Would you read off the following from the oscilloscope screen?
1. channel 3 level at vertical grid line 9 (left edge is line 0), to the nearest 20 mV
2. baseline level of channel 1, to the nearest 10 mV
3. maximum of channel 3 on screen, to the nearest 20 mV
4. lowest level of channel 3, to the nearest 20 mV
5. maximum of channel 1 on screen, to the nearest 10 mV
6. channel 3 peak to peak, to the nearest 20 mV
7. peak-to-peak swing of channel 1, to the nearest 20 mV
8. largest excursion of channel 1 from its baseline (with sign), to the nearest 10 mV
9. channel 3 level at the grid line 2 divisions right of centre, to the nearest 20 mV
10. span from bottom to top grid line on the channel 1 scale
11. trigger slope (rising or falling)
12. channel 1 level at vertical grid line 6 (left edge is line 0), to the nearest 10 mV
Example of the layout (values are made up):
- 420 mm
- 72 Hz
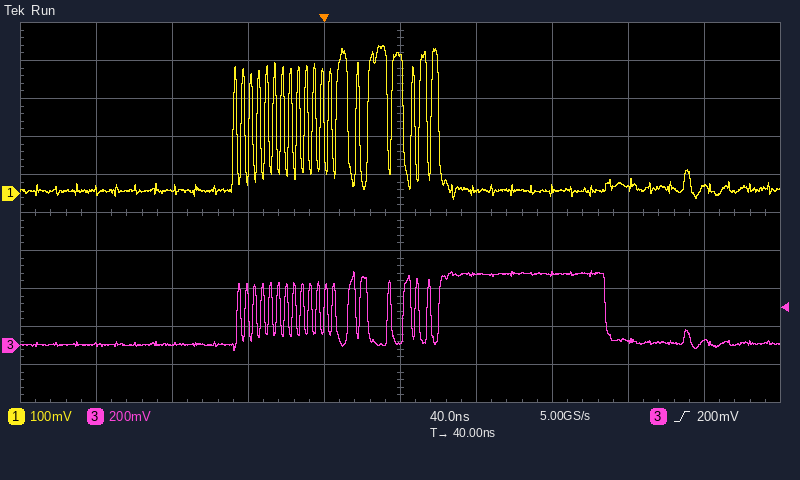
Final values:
- 20 mV
- 10 mV
- 400 mV
- -20 mV
- 390 mV
- 420 mV
- 400 mV
- +380 mV
- 380 mV
- 1 V
- rising
- 10 mV
